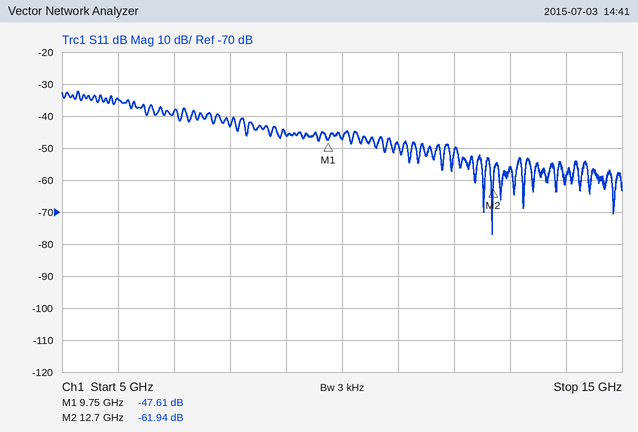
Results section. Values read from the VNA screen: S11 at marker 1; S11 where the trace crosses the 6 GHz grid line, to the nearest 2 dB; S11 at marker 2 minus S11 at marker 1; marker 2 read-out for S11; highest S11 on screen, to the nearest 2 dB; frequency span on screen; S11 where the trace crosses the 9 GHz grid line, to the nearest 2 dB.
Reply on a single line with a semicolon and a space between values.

-47.61 dB; -34 dB; -14.33 dB; -61.94 dB; -32 dB; 10 GHz; -46 dB
